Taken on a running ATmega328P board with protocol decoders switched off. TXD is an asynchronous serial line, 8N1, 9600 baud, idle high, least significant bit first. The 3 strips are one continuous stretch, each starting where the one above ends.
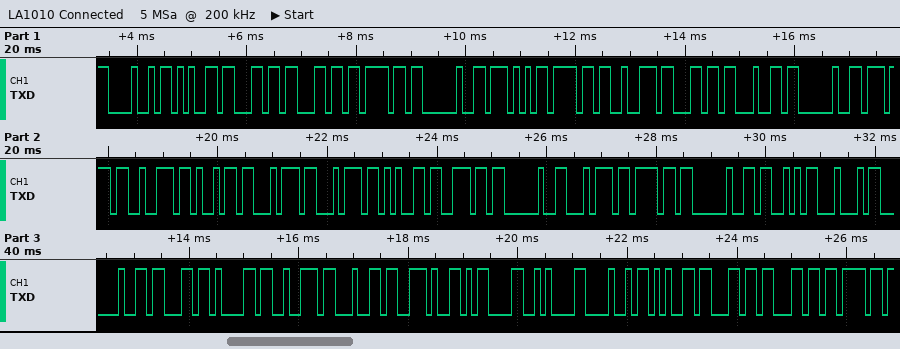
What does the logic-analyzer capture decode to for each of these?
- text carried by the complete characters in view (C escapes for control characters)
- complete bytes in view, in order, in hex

"Hello World written to SD card.\r\nHello"
48 65 6C 6C 6F 20 57 6F 72 6C 64 20 77 72 69 74 74 65 6E 20 74 6F 20 53 44 20 63 61 72 64 2E 0D 0A 48 65 6C 6C 6F
